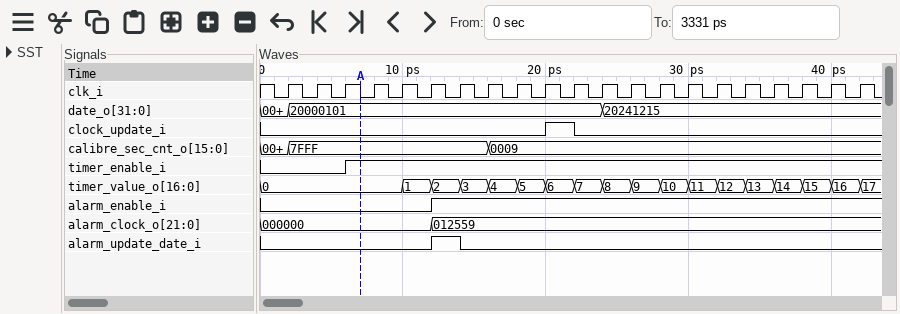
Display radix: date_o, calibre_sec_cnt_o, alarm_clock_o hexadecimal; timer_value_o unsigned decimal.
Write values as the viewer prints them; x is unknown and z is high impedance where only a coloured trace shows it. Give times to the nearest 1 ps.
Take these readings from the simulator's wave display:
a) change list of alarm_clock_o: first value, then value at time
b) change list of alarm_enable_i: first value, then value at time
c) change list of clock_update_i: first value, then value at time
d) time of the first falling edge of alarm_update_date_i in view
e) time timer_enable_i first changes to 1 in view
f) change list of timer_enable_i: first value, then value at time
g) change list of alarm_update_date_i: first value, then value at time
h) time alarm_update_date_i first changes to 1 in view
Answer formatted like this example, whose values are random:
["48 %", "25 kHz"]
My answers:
["000000, 012559 at 12 ps", "0, 1 at 12 ps", "0, 1 at 20 ps, 0 at 22 ps", "14 ps", "6 ps", "0, 1 at 6 ps", "0, 1 at 12 ps, 0 at 14 ps", "12 ps"]
